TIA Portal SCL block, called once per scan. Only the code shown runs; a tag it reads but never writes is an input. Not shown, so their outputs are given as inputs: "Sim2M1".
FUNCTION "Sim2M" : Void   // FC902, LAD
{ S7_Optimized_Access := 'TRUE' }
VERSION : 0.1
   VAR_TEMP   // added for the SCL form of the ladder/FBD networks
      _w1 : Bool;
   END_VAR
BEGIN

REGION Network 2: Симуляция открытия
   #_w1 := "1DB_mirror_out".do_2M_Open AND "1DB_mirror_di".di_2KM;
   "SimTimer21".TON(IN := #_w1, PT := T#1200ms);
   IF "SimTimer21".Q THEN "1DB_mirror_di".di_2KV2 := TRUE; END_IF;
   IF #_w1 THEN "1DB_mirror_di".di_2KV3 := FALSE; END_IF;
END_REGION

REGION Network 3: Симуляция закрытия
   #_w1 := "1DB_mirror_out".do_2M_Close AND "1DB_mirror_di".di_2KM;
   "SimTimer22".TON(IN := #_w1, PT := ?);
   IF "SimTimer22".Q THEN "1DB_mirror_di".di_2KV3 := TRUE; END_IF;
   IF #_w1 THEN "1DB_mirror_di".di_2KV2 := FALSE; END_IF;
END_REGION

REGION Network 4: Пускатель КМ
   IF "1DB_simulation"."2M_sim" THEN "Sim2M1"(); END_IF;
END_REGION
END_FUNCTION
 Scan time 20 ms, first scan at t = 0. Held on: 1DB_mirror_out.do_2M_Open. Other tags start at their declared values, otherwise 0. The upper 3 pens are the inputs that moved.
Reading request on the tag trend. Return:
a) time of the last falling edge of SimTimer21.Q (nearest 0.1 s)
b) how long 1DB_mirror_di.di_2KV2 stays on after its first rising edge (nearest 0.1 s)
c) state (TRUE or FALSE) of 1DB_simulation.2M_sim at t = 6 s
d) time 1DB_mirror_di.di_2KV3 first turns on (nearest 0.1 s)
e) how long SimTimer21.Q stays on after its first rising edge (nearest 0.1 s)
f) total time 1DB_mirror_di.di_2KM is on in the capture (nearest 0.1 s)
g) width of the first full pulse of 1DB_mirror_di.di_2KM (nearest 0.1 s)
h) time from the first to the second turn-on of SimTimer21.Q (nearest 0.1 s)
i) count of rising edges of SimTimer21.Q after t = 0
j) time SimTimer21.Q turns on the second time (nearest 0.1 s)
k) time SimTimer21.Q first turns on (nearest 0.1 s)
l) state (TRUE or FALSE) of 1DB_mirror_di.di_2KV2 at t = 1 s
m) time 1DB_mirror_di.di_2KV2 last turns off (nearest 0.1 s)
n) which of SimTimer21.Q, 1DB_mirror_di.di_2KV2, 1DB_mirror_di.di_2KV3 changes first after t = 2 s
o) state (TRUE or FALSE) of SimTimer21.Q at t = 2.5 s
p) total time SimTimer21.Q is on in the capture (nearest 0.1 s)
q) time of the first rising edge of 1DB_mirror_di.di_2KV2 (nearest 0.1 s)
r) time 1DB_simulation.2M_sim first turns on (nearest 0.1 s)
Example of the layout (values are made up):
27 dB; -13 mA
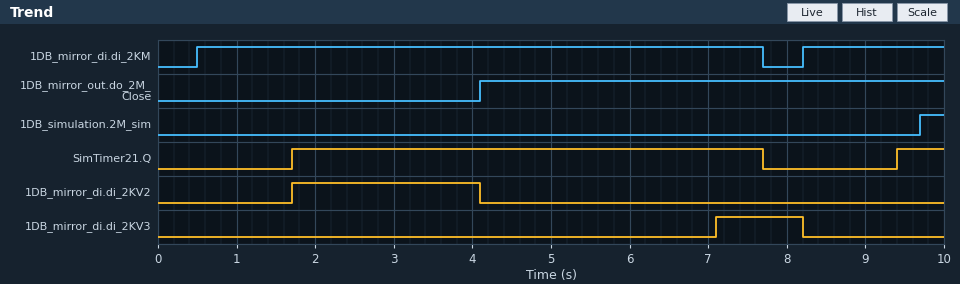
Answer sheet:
7.7 s; 2.4 s; FALSE; 7.1 s; 6.0 s; 9.0 s; 7.2 s; 7.7 s; 2; 9.4 s; 1.7 s; FALSE; 4.1 s; 1DB_mirror_di.di_2KV2; TRUE; 6.6 s; 1.7 s; 9.7 s
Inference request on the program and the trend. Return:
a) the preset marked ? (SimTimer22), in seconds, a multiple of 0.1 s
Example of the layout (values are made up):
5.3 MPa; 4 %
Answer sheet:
3.0 s
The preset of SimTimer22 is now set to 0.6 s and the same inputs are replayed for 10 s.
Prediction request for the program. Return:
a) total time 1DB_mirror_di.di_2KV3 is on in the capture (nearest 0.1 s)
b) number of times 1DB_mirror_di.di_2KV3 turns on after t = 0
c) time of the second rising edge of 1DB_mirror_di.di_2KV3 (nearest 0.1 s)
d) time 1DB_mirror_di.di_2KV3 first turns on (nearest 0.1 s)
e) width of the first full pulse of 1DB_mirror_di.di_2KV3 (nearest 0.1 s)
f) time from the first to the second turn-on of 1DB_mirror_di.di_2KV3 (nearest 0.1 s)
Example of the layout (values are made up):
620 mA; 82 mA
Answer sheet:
4.7 s; 2; 8.8 s; 4.7 s; 3.5 s; 4.1 s
